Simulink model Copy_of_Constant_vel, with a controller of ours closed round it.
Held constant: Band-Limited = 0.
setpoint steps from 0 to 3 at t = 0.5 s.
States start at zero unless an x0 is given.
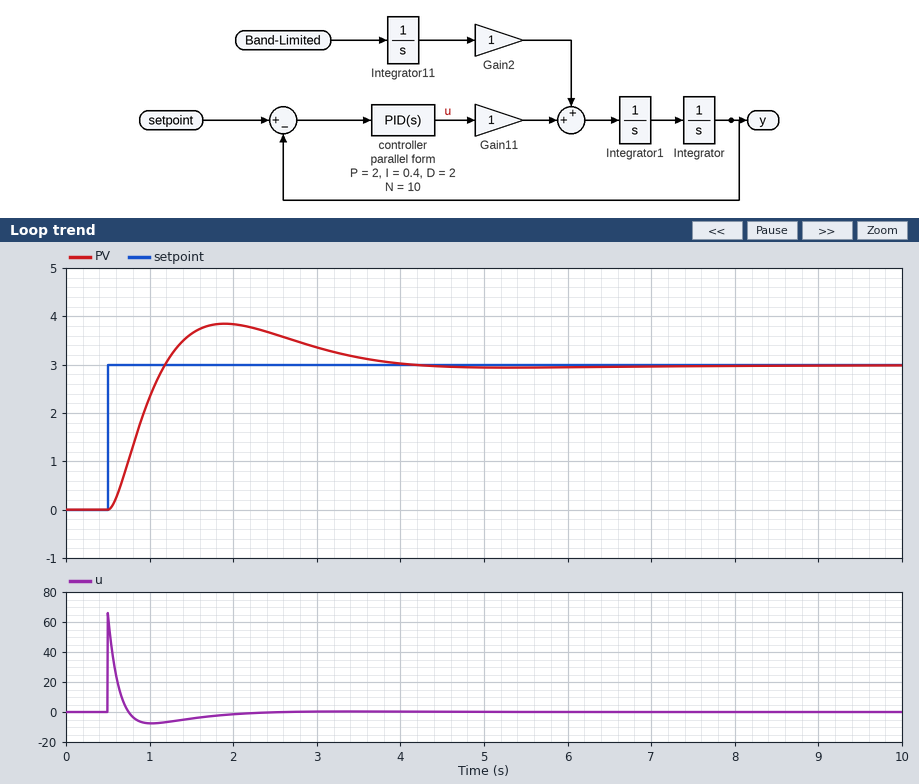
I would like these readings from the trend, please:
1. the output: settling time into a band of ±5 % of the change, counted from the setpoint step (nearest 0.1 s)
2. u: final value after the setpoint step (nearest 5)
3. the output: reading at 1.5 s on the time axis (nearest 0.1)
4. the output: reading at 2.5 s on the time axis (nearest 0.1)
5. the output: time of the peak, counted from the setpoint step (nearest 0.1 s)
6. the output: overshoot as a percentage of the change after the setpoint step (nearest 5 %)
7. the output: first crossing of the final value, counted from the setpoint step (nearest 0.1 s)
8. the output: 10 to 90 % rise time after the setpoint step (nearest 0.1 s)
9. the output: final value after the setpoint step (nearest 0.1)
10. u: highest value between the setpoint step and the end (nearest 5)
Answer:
3.0 s
0
3.6
3.6
1.4 s
30 %
0.7 s
0.5 s
3.0
65
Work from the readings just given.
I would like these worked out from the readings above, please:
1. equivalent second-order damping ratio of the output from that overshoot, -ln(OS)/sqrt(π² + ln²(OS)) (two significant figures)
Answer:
0.36
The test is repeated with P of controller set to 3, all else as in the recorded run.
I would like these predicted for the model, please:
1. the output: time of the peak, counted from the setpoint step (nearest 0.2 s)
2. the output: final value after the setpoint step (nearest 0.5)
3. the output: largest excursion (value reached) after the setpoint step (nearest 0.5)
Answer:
1.2 s
3.0
4.0
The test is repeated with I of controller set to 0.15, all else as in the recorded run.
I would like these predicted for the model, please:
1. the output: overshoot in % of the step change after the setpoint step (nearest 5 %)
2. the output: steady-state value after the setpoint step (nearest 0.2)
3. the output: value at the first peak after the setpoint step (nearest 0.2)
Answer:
25 %
3.0
3.8
